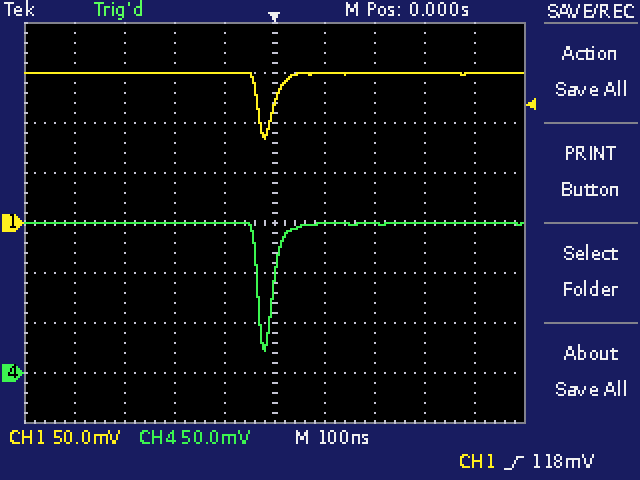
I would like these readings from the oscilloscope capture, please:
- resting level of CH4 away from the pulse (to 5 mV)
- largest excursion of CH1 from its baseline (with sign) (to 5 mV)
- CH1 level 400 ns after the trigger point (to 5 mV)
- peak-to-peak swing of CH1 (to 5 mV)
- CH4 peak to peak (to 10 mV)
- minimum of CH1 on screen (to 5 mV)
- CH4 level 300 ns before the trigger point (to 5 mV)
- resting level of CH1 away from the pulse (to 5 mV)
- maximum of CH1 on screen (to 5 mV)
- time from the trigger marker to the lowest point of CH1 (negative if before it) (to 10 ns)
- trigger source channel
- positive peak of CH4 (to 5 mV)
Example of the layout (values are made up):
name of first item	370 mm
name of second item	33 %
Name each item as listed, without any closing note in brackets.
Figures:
resting level of CH4 away from the pulse	150 mV
largest excursion of CH1 from its baseline (with sign)	-65 mV
CH1 level 400 ns after the trigger point	150 mV
peak-to-peak swing of CH1	65 mV
CH4 peak to peak	130 mV
minimum of CH1 on screen	85 mV
CH4 level 300 ns before the trigger point	150 mV
resting level of CH1 away from the pulse	150 mV
maximum of CH1 on screen	150 mV
time from the trigger marker to the lowest point of CH1 (negative if before it)	-20 ns
trigger source channel	CH1
positive peak of CH4	150 mV
